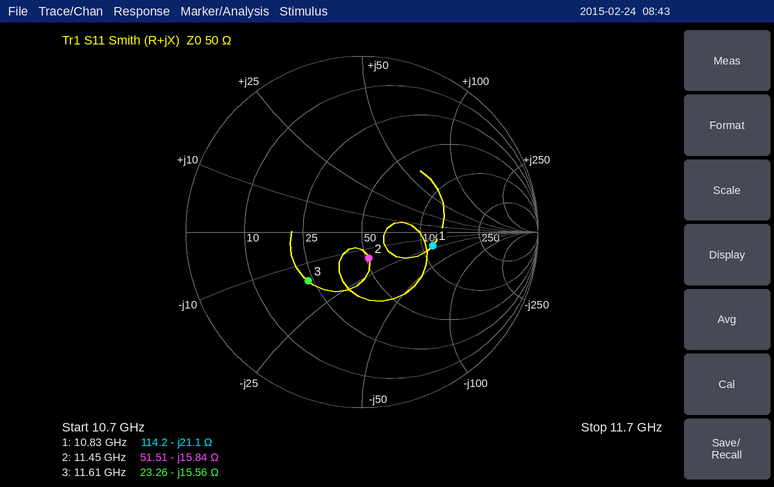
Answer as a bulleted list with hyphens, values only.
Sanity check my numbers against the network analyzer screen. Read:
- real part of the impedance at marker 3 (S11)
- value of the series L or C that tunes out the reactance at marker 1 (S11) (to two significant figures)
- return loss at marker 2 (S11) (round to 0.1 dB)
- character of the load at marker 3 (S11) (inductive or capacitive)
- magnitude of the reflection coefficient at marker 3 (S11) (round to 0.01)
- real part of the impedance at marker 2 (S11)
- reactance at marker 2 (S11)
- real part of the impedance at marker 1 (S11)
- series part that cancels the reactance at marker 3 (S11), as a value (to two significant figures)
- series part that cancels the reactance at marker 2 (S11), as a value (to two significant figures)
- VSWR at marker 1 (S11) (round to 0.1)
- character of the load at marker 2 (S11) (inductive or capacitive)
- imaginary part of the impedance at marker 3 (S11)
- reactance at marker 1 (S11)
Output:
- 23.26 Ω
- 310 pH
- 16.2 dB
- capacitive
- 0.41
- 51.51 Ω
- -15.84 Ω
- 114.2 Ω
- 210 pH
- 220 pH
- 2.4
- capacitive
- -15.56 Ω
- -21.1 Ω
